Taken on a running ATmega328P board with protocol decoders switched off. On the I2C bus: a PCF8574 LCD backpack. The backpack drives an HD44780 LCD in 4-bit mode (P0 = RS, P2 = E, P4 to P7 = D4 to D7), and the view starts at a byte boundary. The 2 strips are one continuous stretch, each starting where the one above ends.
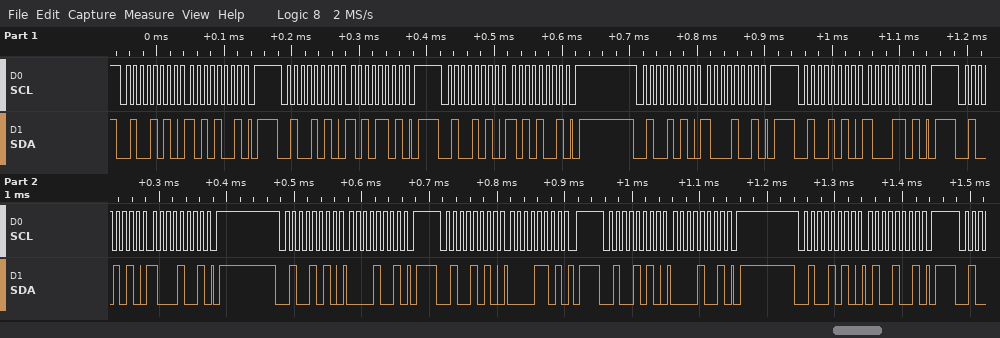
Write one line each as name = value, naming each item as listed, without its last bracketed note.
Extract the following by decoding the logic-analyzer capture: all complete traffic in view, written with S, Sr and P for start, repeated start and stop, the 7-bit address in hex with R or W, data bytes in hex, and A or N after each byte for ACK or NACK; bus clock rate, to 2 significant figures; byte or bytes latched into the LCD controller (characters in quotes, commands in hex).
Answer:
all complete traffic in view, written with S, Sr and P for start, repeated start and stop, the 7-bit address in hex with R or W, data bytes in hex, and A or N after each byte for ACK or NACK = S 25W A A9 A P S 25W A AD A P S 25W A A9 A P S 25W A 89 A P S 25W A 8D A P S 25W A 89 A P S 25W A 09 A P S 25W A 0D A P S 25W A 09 A P S 25W A 49 A P
bus clock rate, to 2 significant figures = 100 kHz
byte or bytes latched into the LCD controller = data 0xA8
